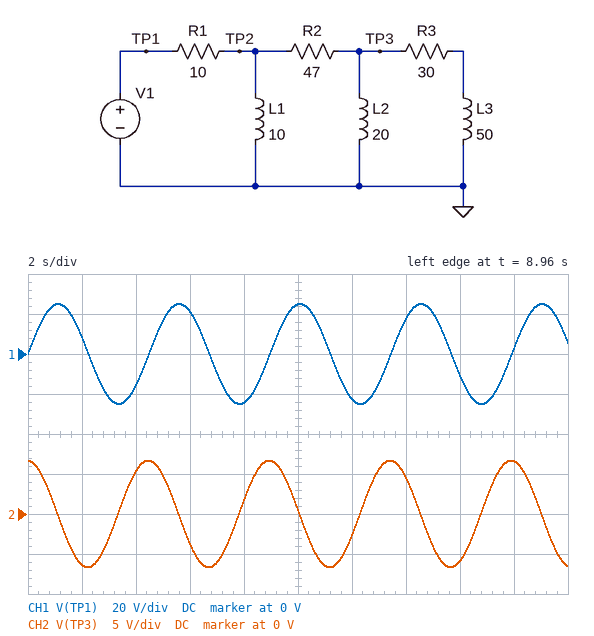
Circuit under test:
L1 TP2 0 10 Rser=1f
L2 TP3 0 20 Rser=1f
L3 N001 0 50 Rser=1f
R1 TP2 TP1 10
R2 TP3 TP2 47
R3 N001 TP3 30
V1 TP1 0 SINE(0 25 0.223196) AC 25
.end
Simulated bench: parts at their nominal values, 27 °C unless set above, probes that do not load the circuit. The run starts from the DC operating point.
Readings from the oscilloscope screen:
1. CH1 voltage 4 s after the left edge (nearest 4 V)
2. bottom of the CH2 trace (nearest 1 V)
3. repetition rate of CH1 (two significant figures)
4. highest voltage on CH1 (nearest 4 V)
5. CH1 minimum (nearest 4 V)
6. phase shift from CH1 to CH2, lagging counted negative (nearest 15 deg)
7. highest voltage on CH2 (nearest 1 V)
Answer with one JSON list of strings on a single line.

["-16 V", "-7 V", "220 mHz", "24 V", "-24 V", "90 deg", "7 V"]
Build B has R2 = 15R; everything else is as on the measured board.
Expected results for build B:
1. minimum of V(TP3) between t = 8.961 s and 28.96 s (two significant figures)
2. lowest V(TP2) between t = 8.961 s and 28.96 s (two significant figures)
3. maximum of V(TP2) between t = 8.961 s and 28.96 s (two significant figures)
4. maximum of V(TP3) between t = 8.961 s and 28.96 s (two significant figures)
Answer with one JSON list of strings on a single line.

["-12 V", "-15 V", "15 V", "12 V"]
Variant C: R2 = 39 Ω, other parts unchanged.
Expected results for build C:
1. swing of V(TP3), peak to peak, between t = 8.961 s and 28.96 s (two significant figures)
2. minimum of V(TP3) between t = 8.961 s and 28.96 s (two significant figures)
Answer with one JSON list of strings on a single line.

["15 V", "-7.5 V"]
